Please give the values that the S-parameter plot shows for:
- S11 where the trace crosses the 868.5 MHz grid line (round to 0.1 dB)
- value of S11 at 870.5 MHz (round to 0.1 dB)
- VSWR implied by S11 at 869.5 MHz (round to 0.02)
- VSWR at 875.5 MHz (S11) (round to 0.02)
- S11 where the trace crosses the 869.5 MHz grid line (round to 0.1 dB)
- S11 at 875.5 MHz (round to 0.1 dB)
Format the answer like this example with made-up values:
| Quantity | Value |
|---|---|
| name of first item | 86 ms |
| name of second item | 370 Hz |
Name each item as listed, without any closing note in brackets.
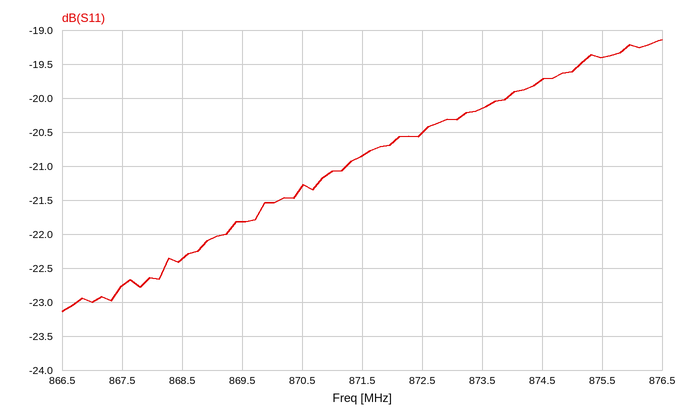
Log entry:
| Quantity | Value |
|---|---|
| S11 where the trace crosses the 868.5 MHz grid line | -22.4 dB |
| value of S11 at 870.5 MHz | -21.3 dB |
| VSWR implied by S11 at 869.5 MHz | 1.18 |
| VSWR at 875.5 MHz (S11) | 1.24 |
| S11 where the trace crosses the 869.5 MHz grid line | -21.8 dB |
| S11 at 875.5 MHz | -19.4 dB |
